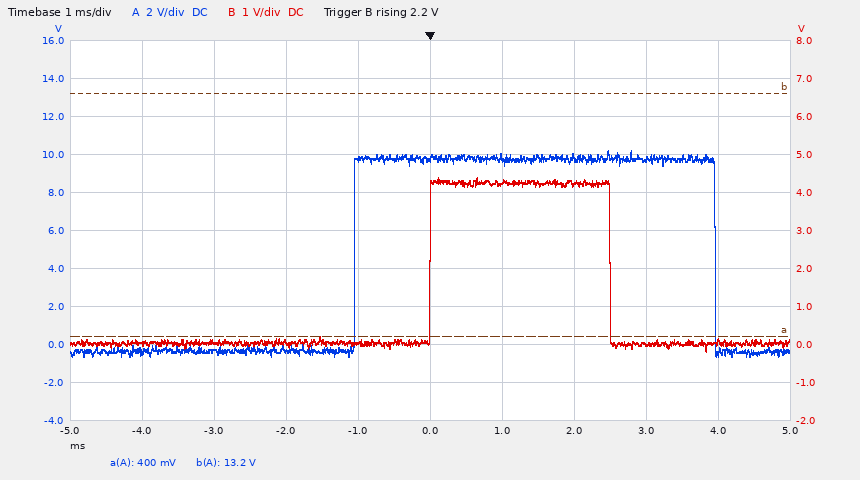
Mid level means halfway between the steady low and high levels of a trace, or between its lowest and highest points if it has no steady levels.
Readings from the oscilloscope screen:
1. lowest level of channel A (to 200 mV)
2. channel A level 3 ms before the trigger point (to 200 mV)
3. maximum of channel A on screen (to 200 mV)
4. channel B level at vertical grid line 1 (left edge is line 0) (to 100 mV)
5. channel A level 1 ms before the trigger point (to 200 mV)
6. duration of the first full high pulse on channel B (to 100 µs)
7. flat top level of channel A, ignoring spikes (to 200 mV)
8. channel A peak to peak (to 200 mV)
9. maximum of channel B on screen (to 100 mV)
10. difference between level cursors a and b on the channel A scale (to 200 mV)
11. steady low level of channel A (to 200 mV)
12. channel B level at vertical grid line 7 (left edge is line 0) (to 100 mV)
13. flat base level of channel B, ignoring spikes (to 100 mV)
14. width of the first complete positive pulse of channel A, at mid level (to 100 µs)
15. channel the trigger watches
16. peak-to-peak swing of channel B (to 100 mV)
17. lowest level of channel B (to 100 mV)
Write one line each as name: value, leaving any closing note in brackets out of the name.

lowest level of channel A: -600 mV
channel A level 3 ms before the trigger point: -400 mV
maximum of channel A on screen: 10.2 V
channel B level at vertical grid line 1 (left edge is line 0): 0.0 V
channel A level 1 ms before the trigger point: 9.8 V
duration of the first full high pulse on channel B: 2.5 ms
flat top level of channel A, ignoring spikes: 9.8 V
channel A peak to peak: 10.8 V
maximum of channel B on screen: 4.4 V
difference between level cursors a and b on the channel A scale: 12.8 V
steady low level of channel A: -400 mV
channel B level at vertical grid line 7 (left edge is line 0): 4.2 V
flat base level of channel B, ignoring spikes: 0.0 V
width of the first complete positive pulse of channel A, at mid level: 5.0 ms
channel the trigger watches: channel B
peak-to-peak swing of channel B: 4.6 V
lowest level of channel B: -200 mV
